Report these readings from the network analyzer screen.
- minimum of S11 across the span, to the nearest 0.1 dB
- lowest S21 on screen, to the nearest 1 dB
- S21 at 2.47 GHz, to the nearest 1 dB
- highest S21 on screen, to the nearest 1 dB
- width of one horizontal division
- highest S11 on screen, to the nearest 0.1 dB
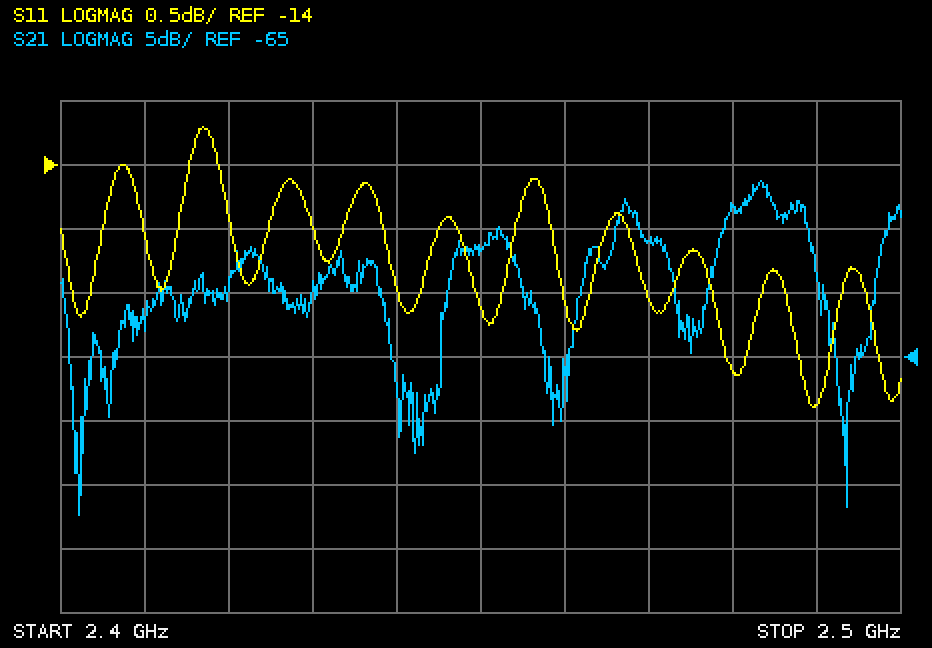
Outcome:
-15.9 dB
-77 dB
-56 dB
-51 dB
10 MHz
-13.7 dB
